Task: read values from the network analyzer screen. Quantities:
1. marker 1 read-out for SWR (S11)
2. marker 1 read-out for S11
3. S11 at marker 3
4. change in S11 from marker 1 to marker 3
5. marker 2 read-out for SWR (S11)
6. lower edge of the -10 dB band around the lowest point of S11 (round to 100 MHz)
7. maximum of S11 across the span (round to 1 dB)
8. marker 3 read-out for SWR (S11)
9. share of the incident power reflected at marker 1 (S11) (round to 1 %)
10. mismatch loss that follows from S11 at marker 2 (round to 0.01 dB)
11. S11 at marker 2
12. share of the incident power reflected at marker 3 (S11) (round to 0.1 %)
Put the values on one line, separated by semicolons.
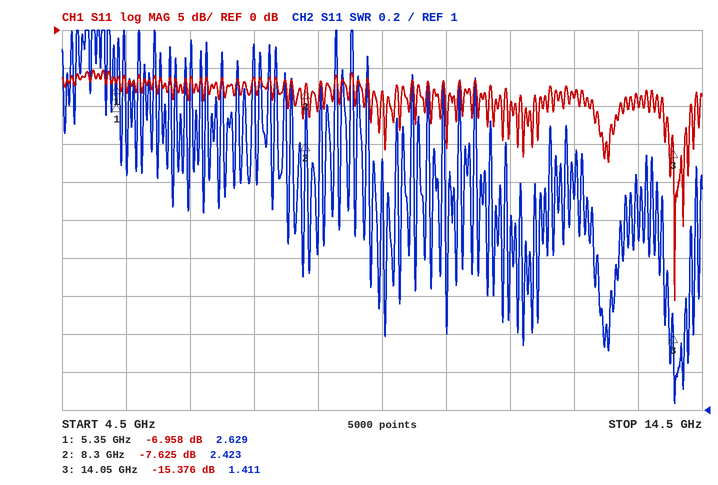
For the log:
2.629; -6.958 dB; -15.376 dB; -8.418 dB; 2.423; 13.9 GHz; -5 dB; 1.411; 20 %; 0.82 dB; -7.625 dB; 2.9 %
